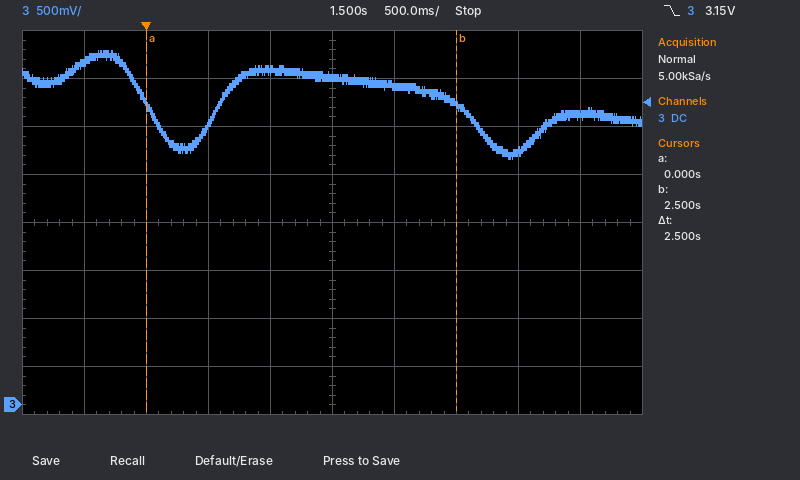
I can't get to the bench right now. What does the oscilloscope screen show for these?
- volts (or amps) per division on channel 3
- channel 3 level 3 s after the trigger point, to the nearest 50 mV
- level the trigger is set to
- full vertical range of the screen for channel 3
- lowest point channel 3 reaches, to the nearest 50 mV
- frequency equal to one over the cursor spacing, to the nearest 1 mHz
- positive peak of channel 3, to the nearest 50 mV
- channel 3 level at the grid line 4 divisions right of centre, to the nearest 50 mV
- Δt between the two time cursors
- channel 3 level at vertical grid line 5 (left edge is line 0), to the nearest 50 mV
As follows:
500 mV
2.65 V
3.15 V
4 V
2.55 V
400 mHz
3.70 V
3.00 V
2.5 s
3.40 V
